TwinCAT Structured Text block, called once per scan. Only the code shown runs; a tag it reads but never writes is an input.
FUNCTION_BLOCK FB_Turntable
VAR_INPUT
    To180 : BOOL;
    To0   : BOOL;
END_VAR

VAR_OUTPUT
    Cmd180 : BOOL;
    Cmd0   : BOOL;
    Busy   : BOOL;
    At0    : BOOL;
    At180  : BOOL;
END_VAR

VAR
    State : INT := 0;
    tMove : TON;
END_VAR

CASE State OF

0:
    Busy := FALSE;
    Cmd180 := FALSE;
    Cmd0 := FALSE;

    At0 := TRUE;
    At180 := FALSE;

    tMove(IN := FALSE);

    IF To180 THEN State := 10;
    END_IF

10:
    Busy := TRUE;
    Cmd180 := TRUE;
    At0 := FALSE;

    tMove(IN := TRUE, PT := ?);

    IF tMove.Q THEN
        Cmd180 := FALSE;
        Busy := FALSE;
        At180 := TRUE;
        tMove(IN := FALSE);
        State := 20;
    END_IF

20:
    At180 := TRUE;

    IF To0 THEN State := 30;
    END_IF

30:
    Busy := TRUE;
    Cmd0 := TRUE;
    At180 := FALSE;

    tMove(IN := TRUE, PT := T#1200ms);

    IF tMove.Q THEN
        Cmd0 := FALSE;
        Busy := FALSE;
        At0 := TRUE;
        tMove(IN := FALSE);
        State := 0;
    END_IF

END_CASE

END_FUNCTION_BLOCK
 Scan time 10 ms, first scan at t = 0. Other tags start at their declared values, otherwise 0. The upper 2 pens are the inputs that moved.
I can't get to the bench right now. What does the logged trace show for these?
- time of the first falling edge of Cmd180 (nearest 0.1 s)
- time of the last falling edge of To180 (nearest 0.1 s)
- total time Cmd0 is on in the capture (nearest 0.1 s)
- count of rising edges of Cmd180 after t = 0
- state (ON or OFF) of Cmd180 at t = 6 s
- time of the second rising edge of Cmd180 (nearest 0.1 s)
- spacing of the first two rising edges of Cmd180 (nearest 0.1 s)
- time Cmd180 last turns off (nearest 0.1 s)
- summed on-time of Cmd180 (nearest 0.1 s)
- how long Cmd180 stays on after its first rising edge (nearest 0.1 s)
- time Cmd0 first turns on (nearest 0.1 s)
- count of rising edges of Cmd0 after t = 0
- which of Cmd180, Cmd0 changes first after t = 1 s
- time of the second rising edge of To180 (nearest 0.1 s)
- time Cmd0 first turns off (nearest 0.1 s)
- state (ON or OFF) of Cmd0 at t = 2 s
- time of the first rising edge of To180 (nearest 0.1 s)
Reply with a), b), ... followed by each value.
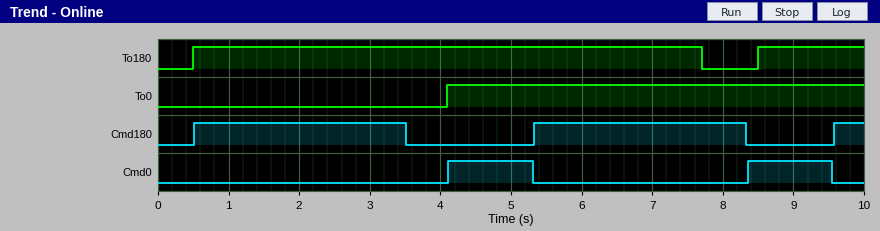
a) 3.5 s
b) 7.7 s
c) 2.4 s
d) 3
e) ON
f) 5.3 s
g) 4.8 s
h) 8.3 s
i) 6.4 s
j) 3.0 s
k) 4.1 s
l) 2
m) Cmd180
n) 8.5 s
o) 5.3 s
p) OFF
q) 0.5 s
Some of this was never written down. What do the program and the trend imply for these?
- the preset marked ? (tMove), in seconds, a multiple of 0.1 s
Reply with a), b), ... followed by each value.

a) 3.0 s
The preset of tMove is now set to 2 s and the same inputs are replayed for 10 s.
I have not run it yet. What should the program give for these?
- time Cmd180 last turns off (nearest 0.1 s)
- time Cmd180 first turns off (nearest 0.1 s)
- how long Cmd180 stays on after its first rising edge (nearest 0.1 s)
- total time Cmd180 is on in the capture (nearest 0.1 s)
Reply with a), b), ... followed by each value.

a) 7.3 s
b) 2.5 s
c) 2.0 s
d) 5.4 s
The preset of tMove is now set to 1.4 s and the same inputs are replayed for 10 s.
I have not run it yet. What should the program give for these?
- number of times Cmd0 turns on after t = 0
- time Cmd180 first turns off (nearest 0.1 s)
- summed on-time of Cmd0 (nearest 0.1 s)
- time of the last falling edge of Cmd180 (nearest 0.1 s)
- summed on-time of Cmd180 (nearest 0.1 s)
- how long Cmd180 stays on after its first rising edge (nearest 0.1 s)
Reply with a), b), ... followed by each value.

a) 3
b) 1.9 s
c) 2.5 s
d) 9.9 s
e) 4.2 s
f) 1.4 s
